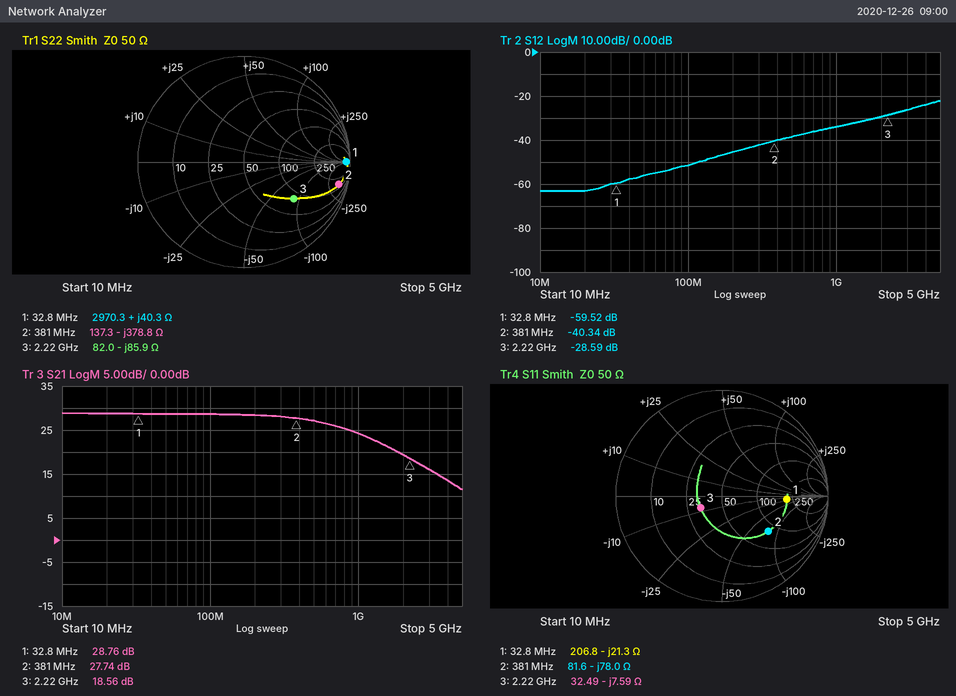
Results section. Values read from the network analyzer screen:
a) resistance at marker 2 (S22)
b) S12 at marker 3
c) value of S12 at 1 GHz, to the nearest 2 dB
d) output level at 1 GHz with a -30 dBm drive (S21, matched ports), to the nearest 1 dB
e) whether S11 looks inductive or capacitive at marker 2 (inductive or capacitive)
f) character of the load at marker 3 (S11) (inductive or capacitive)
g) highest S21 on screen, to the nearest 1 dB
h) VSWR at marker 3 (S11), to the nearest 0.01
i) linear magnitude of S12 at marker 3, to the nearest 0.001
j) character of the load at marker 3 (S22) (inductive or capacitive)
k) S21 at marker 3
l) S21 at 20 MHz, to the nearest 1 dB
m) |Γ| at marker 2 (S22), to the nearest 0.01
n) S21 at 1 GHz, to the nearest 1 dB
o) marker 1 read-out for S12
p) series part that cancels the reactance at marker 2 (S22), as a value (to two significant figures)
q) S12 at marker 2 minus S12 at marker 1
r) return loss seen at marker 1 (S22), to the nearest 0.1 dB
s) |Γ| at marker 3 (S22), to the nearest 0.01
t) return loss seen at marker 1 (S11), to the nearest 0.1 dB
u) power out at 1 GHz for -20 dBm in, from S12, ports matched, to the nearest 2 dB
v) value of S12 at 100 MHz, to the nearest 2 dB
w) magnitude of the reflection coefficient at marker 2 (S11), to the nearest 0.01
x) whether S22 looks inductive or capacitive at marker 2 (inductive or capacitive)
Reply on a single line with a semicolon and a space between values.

137.3 Ω; -28.59 dB; -34 dB; -6 dBm; capacitive; capacitive; 29 dB; 1.60; 0.037; capacitive; 18.56 dB; 29 dB; 0.92; 24 dB; -59.52 dB; 160 nH; 19.18 dB; 0.3 dB; 0.58; 4.2 dB; -54 dBm; -52 dB; 0.55; capacitive
